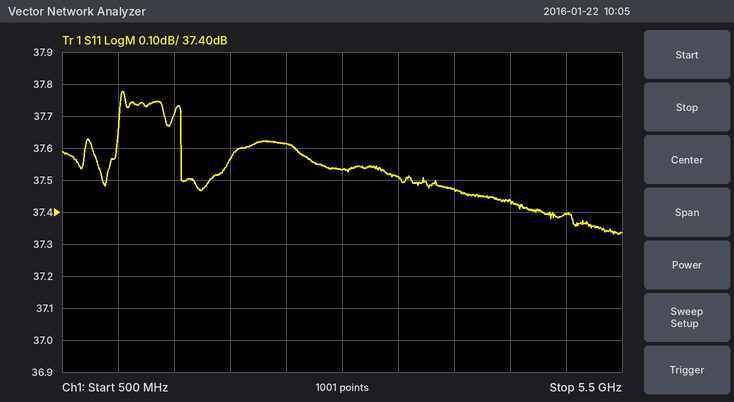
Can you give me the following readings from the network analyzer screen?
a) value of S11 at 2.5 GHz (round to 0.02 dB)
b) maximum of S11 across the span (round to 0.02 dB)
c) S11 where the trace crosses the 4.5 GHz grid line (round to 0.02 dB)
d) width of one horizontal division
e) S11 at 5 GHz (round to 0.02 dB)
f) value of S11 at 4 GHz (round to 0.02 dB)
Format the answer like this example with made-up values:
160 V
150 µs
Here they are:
37.62 dB
37.78 dB
37.44 dB
500 MHz
37.40 dB
37.48 dB
